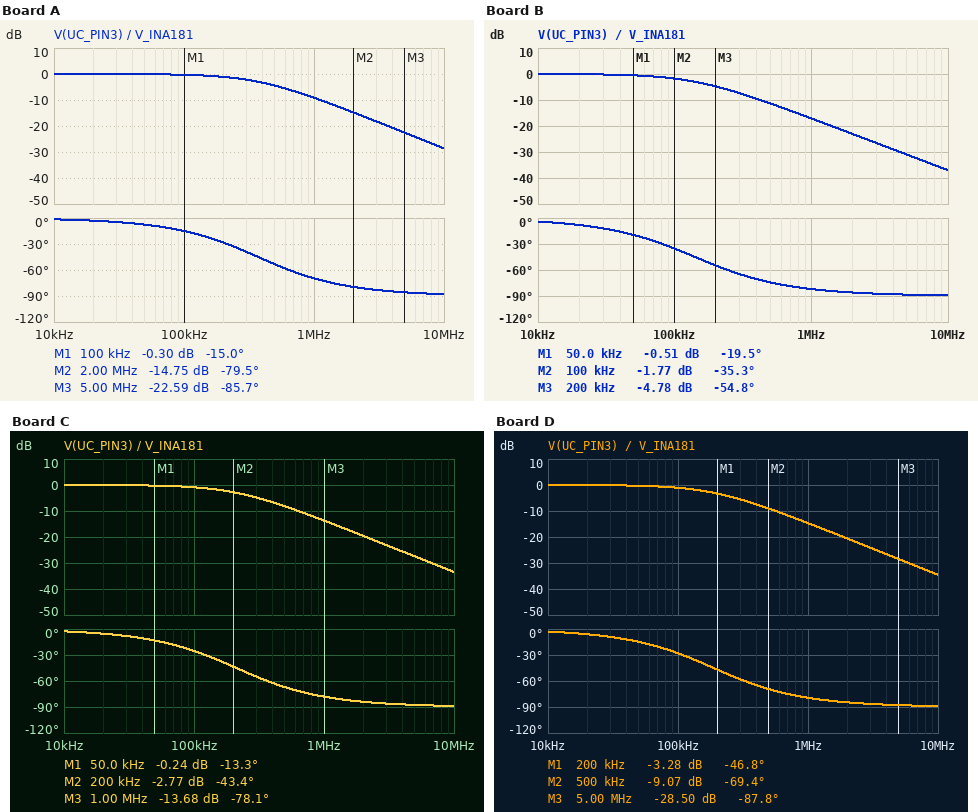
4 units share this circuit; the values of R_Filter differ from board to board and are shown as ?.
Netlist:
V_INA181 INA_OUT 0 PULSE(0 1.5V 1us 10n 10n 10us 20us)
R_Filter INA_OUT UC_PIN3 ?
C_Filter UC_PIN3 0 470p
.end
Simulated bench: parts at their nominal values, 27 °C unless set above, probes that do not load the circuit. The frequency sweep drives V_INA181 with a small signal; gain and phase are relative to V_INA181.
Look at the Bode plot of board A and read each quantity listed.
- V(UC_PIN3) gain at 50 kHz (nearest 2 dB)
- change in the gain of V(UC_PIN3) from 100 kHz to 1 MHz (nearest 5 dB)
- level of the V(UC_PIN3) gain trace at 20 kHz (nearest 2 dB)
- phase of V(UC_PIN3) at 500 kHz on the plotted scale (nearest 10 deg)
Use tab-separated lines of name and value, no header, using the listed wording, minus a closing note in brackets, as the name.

V(UC_PIN3) gain at 50 kHz	0 dB
change in the gain of V(UC_PIN3) from 100 kHz to 1 MHz	-10 dB
level of the V(UC_PIN3) gain trace at 20 kHz	0 dB
phase of V(UC_PIN3) at 500 kHz on the plotted scale	-50 deg
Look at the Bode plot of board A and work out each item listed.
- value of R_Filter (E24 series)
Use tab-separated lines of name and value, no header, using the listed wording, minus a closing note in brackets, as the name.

value of R_Filter	910 Ω
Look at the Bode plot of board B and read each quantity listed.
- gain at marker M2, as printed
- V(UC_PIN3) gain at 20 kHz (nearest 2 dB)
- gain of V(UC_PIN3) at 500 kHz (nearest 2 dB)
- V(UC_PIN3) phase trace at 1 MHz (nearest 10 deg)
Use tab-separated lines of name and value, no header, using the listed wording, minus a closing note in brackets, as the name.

gain at marker M2, as printed	-1.77 dB
V(UC_PIN3) gain at 20 kHz	0 dB
gain of V(UC_PIN3) at 500 kHz	-12 dB
V(UC_PIN3) phase trace at 1 MHz	-80 deg
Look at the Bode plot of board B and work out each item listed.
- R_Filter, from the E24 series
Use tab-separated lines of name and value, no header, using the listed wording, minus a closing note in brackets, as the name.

R_Filter, from the E24 series	2.4 kΩ
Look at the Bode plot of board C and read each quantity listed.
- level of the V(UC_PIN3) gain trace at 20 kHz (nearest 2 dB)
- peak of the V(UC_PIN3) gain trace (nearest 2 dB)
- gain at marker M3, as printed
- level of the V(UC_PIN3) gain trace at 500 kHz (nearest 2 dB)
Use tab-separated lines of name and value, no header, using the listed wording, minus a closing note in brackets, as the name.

level of the V(UC_PIN3) gain trace at 20 kHz	0 dB
peak of the V(UC_PIN3) gain trace	0 dB
gain at marker M3, as printed	-13.68 dB
level of the V(UC_PIN3) gain trace at 500 kHz	-8 dB
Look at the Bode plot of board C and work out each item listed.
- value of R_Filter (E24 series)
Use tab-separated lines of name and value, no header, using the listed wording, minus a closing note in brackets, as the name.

value of R_Filter	1.6 kΩ
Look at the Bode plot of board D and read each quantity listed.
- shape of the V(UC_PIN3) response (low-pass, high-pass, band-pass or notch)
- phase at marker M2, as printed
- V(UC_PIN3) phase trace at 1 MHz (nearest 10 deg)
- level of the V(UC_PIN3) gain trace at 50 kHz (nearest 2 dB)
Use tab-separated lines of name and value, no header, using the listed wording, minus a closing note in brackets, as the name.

shape of the V(UC_PIN3) response	low-pass
phase at marker M2, as printed	-69.4 deg
V(UC_PIN3) phase trace at 1 MHz	-80 deg
level of the V(UC_PIN3) gain trace at 50 kHz	0 dB
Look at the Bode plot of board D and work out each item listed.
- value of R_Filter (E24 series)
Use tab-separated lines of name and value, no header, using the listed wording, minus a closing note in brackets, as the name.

value of R_Filter	1.8 kΩ
